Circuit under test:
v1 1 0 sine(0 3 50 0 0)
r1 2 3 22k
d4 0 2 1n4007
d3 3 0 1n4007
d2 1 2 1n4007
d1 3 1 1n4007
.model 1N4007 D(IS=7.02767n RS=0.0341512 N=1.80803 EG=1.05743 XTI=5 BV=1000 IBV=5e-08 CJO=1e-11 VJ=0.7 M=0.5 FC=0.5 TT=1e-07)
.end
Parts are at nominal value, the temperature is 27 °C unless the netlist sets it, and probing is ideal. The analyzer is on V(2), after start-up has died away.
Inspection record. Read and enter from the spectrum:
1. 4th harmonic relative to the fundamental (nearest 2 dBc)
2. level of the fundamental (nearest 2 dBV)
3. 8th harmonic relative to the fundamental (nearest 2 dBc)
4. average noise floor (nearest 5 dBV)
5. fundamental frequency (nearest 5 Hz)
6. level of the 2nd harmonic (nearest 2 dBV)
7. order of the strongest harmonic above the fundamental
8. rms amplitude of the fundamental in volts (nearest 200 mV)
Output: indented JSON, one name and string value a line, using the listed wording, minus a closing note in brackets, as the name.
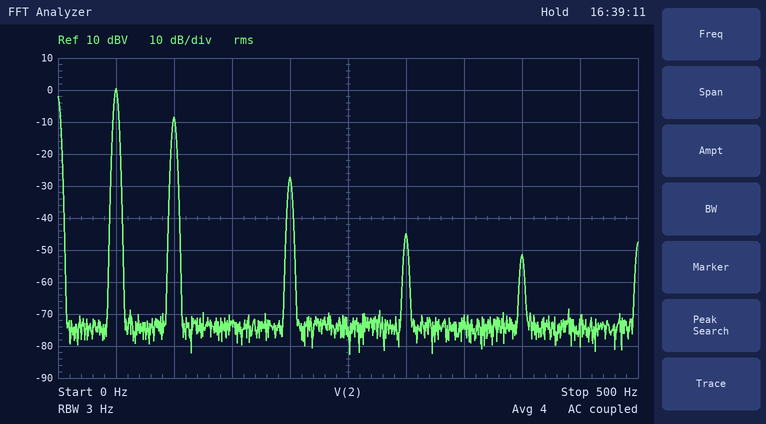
{
  "4th harmonic relative to the fundamental": "-28 dBc",
  "level of the fundamental": "0 dBV",
  "8th harmonic relative to the fundamental": "-52 dBc",
  "average noise floor": "-75 dBV",
  "fundamental frequency": "50 Hz",
  "level of the 2nd harmonic": "-8 dBV",
  "order of the strongest harmonic above the fundamental": "2",
  "rms amplitude of the fundamental in volts": "1.0 V"
}
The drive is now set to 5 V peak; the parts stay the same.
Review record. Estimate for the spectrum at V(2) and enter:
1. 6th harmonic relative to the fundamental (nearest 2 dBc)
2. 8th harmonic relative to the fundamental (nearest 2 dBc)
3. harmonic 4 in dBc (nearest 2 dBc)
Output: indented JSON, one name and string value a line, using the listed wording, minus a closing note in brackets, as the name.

{
  "6th harmonic relative to the fundamental": "-34 dBc",
  "8th harmonic relative to the fundamental": "-44 dBc",
  "harmonic 4 in dBc": "-24 dBc"
}
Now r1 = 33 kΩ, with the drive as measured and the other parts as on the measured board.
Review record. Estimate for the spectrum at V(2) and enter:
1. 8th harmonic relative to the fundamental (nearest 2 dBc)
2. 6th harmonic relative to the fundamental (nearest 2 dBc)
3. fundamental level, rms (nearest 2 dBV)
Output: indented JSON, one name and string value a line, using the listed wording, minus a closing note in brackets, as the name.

{
  "8th harmonic relative to the fundamental": "-58 dBc",
  "6th harmonic relative to the fundamental": "-42 dBc",
  "fundamental level, rms": "0 dBV"
}
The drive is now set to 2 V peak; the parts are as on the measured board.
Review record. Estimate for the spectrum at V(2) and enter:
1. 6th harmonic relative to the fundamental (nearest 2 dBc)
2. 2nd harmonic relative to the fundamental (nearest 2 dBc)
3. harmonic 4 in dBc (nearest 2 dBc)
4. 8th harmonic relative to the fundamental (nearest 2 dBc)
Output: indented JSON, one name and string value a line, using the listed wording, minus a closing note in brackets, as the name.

{
  "6th harmonic relative to the fundamental": "-42 dBc",
  "2nd harmonic relative to the fundamental": "-10 dBc",
  "harmonic 4 in dBc": "-36 dBc",
  "8th harmonic relative to the fundamental": "-42 dBc"
}
